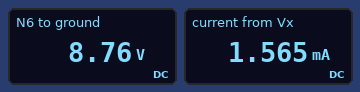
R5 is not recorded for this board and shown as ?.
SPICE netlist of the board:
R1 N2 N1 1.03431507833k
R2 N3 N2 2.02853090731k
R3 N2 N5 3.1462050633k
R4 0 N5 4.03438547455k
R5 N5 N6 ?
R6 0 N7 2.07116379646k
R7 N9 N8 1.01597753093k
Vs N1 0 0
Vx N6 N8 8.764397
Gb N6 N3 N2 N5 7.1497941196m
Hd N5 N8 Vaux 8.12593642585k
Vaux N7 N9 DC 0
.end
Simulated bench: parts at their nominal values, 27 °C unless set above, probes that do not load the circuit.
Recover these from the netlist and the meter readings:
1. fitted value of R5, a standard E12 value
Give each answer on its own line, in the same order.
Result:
5.6 kΩ
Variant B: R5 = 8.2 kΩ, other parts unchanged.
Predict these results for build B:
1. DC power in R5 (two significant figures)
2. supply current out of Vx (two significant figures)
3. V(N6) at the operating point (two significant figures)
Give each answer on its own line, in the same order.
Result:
9.4 mW
1.1 mA
8.8 V
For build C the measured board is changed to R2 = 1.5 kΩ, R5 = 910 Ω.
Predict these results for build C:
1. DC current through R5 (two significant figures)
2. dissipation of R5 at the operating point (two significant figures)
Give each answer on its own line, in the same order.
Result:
9.6 mA
84 mW
